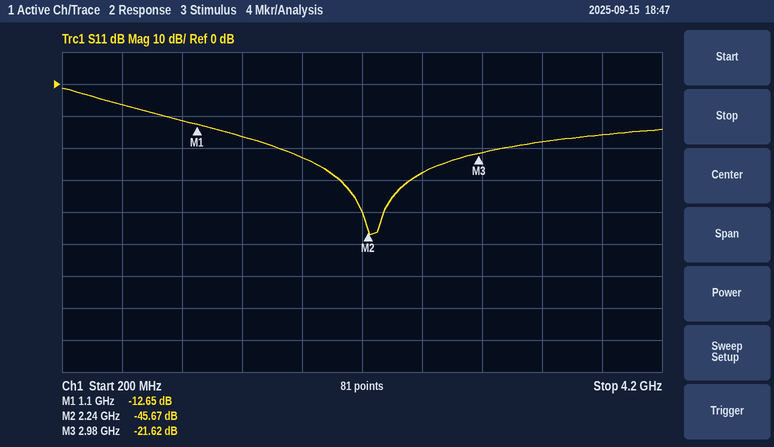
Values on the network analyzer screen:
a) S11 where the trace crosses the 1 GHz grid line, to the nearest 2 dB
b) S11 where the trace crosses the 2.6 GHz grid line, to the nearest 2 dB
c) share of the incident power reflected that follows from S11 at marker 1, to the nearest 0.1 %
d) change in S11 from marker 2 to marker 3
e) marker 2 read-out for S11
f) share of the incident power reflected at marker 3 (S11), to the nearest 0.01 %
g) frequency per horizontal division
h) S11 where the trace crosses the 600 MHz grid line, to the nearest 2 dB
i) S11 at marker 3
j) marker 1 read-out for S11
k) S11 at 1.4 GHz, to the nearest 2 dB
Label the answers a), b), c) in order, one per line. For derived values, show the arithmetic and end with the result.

a) -12 dB
b) -28 dB
c) 10^(-12.65/10) ≈ 5.4 %
d) -21.62 − (-45.67) = 24.05 dB
e) -45.67 dB
f) 10^(-21.62/10) ≈ 0.69 %
g) 400 MHz
h) -6 dB
i) -21.62 dB
j) -12.65 dB
k) -16 dB
